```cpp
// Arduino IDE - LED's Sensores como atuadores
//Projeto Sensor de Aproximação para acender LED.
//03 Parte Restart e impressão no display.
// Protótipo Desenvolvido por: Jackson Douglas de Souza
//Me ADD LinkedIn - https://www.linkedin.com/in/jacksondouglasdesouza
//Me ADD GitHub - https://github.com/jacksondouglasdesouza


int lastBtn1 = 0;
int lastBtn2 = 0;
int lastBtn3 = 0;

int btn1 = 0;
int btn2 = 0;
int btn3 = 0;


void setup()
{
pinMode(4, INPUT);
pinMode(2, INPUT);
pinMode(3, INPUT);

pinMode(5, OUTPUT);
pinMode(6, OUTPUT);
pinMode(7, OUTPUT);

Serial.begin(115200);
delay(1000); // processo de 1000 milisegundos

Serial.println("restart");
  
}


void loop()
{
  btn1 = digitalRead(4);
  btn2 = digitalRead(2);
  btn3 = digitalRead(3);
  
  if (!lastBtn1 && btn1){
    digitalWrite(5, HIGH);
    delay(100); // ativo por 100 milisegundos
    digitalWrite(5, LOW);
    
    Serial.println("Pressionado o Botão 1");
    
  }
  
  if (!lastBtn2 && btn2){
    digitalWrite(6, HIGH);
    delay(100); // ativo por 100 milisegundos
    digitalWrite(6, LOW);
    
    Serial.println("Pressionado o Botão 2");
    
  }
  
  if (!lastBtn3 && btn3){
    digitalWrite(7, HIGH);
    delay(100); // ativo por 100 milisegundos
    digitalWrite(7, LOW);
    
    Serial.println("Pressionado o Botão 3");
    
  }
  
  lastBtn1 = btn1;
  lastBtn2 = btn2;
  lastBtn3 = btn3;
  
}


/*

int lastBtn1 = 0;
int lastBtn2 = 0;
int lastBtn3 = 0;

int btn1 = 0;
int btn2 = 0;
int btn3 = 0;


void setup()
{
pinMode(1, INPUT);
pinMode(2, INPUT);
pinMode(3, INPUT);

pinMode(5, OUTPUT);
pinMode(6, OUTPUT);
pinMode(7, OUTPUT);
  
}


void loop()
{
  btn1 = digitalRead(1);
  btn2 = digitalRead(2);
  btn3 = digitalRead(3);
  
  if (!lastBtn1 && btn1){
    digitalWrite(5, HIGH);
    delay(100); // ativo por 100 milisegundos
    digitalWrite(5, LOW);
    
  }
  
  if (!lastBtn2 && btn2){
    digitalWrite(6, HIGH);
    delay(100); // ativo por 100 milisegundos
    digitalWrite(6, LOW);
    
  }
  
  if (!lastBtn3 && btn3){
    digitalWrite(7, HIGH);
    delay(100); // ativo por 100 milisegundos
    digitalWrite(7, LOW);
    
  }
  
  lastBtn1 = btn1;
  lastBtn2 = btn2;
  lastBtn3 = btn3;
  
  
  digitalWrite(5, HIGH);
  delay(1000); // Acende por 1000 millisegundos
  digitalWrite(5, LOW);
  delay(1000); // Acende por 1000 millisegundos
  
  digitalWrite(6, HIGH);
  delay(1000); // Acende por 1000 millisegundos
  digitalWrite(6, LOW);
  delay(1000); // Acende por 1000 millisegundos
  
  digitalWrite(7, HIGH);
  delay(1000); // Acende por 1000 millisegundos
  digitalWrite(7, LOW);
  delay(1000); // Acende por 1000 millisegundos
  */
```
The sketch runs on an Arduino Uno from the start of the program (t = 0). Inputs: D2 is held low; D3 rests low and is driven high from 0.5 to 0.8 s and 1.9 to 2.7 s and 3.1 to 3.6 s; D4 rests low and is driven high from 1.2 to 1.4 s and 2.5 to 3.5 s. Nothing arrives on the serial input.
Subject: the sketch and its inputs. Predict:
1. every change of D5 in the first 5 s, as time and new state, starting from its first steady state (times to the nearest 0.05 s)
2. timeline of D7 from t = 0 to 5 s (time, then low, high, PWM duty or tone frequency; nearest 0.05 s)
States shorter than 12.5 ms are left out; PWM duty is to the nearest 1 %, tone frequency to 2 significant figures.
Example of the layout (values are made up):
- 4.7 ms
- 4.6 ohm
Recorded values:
- 0 s low; 1.2 s high; 1.3 s low; 2.5 s high; 2.6 s low
- 0 s low; 1.9 s high; 2 s low; 3.1 s high; 3.2 s low
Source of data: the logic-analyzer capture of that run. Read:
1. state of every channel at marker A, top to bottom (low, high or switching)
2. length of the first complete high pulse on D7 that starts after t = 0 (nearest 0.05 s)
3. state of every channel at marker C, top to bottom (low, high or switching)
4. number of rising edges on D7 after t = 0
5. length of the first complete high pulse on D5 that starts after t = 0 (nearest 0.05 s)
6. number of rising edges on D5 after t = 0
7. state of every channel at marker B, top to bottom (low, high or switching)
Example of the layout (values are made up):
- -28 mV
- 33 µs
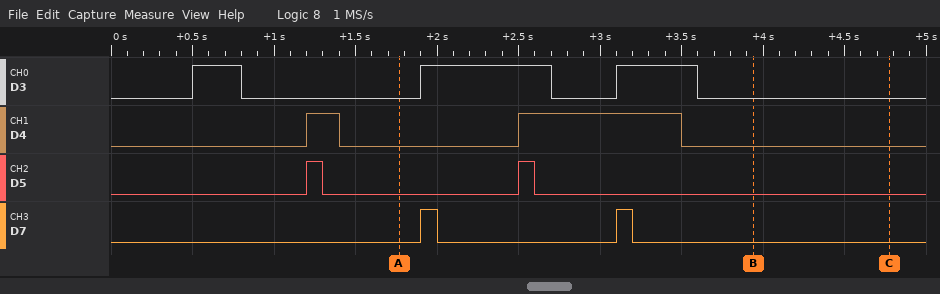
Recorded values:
- D3 low, D4 low, D5 low, D7 low
- 0.10 s
- D3 low, D4 low, D5 low, D7 low
- 2
- 0.10 s
- 2
- D3 low, D4 low, D5 low, D7 low
